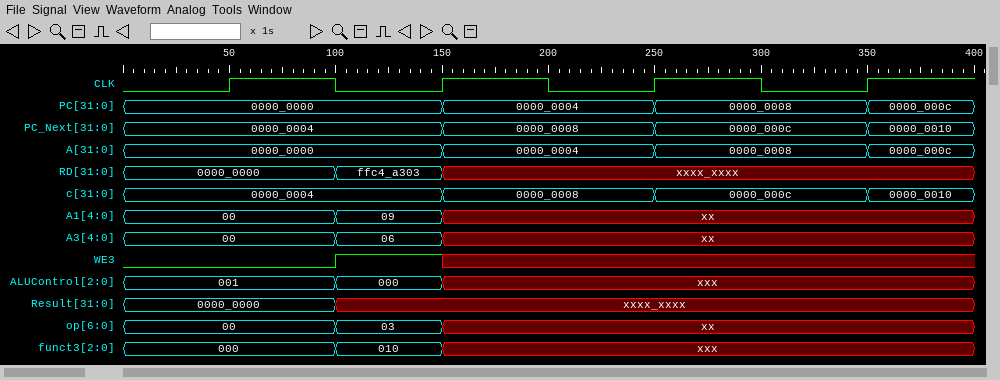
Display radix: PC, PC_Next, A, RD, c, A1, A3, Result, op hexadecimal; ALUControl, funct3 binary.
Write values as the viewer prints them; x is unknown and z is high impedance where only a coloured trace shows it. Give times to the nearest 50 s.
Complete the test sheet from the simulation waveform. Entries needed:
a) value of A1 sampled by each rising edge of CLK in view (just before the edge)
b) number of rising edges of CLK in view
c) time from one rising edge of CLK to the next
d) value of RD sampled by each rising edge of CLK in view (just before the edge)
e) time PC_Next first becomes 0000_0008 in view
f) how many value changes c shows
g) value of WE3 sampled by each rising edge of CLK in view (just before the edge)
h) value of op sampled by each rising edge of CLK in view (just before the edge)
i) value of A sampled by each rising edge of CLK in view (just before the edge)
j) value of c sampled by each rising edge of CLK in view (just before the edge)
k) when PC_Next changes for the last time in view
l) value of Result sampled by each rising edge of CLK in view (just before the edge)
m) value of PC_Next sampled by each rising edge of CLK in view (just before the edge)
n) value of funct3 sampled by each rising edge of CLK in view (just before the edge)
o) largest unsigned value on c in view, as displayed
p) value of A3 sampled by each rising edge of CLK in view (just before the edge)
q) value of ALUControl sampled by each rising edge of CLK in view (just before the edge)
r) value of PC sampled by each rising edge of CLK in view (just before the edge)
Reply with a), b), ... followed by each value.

a) 00, 09, xx, xx
b) 4
c) 100 s
d) 0000_0000, ffc4_a303, xxxx_xxxx, xxxx_xxxx
e) 150 s
f) 3
g) 0 1 x x
h) 00, 03, xx, xx
i) 0000_0000, 0000_0000, 0000_0004, 0000_0008
j) 0000_0004, 0000_0004, 0000_0008, 0000_000c
k) 350 s
l) 0000_0000, xxxx_xxxx, xxxx_xxxx, xxxx_xxxx
m) 0000_0004, 0000_0004, 0000_0008, 0000_000c
n) 000, 010, xxx, xxx
o) 0000_0010
p) 00, 06, xx, xx
q) 001, 000, xxx, xxx
r) 0000_0000, 0000_0000, 0000_0004, 0000_0008
